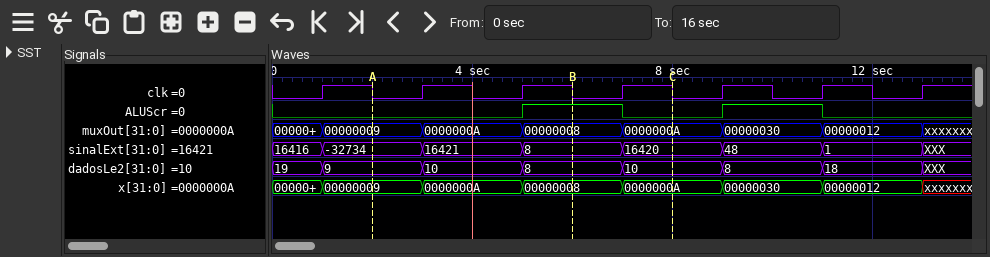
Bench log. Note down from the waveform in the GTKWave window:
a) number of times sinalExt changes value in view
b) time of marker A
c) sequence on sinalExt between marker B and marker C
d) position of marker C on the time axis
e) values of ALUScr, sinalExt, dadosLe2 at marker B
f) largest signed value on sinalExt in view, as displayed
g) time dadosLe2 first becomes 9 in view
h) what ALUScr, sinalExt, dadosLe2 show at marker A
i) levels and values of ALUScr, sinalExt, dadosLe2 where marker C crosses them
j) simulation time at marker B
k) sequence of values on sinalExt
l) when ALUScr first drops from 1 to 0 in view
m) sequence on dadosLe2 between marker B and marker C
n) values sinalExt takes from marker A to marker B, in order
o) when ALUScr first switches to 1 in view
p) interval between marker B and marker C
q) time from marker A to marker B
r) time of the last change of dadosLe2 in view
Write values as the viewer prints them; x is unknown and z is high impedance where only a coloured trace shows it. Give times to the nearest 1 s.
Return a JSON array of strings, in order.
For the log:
["7", "2 s", "8, 16420", "8 s", "ALUScr=1, sinalExt=8, dadosLe2=8", "16421", "1 s", "ALUScr=0, sinalExt=-32734, dadosLe2=9", "ALUScr=0, sinalExt=16420, dadosLe2=10", "6 s", "16416, -32734, 16421, 8, 16420, 48, 1, XXX", "7 s", "8, 10", "-32734, 16421, 8", "5 s", "2 s", "4 s", "13 s"]
